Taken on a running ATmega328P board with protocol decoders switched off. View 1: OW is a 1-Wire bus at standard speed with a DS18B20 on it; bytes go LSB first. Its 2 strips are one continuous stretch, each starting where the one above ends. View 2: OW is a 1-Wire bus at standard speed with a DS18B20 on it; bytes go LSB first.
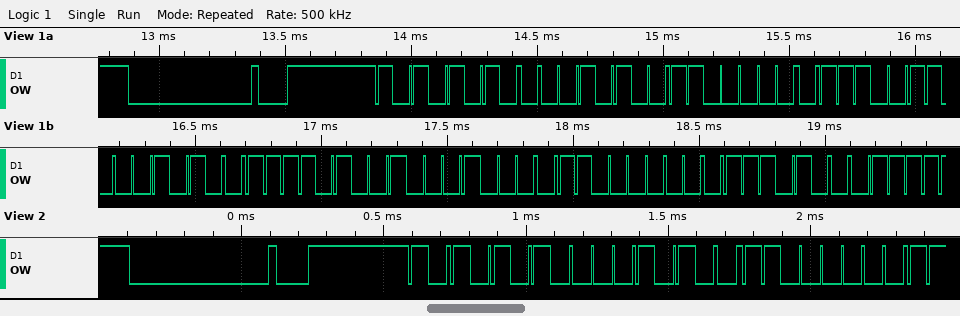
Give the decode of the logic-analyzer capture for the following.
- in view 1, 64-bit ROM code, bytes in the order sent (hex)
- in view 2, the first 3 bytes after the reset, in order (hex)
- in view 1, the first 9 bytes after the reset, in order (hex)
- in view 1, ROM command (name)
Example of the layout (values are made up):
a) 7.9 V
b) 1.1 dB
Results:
a) 28 03 67 94 97 08 03 2E
b) 55 28 03
c) 55 28 03 67 94 97 08 03 2E
d) Match ROM
